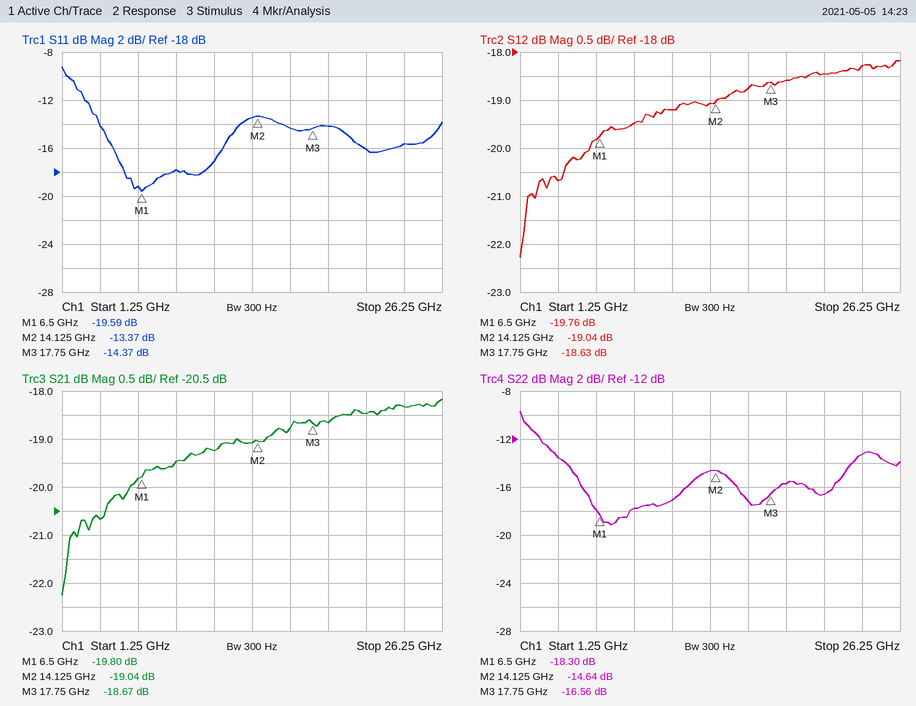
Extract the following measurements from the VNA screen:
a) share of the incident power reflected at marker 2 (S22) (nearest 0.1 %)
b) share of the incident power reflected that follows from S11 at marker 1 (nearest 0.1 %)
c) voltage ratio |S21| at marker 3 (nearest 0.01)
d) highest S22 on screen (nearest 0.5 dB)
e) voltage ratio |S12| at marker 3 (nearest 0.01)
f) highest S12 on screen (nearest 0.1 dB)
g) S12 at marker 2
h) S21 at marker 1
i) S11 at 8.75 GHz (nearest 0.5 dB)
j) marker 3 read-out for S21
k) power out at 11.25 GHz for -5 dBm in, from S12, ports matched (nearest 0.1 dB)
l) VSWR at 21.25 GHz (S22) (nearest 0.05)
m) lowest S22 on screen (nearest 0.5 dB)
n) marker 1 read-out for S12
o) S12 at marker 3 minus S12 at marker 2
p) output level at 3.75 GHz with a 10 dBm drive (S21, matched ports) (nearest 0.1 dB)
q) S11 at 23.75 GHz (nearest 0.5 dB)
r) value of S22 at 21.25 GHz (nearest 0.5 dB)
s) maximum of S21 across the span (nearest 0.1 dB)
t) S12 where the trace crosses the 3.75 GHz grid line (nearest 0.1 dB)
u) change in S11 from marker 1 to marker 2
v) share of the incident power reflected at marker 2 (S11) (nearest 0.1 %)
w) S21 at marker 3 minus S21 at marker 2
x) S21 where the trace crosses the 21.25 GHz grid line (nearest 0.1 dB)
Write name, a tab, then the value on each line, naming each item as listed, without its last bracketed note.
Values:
share of the incident power reflected at marker 2 (S22)	3.4 %
share of the incident power reflected that follows from S11 at marker 1	1.1 %
voltage ratio |S21| at marker 3	0.12
highest S22 on screen	-9.5 dB
voltage ratio |S12| at marker 3	0.12
highest S12 on screen	-18.2 dB
S12 at marker 2	-19.04 dB
S21 at marker 1	-19.80 dB
S11 at 8.75 GHz	-18.0 dB
marker 3 read-out for S21	-18.67 dB
power out at 11.25 GHz for -5 dBm in, from S12, ports matched	-24.2 dBm
VSWR at 21.25 GHz (S22)	1.35
lowest S22 on screen	-19.0 dB
marker 1 read-out for S12	-19.76 dB
S12 at marker 3 minus S12 at marker 2	0.41 dB
output level at 3.75 GHz with a 10 dBm drive (S21, matched ports)	-10.7 dBm
S11 at 23.75 GHz	-15.5 dB
value of S22 at 21.25 GHz	-16.5 dB
maximum of S21 across the span	-18.2 dB
S12 where the trace crosses the 3.75 GHz grid line	-20.7 dB
change in S11 from marker 1 to marker 2	6.22 dB
share of the incident power reflected at marker 2 (S11)	4.6 %
S21 at marker 3 minus S21 at marker 2	0.37 dB
S21 where the trace crosses the 21.25 GHz grid line	-18.5 dB
